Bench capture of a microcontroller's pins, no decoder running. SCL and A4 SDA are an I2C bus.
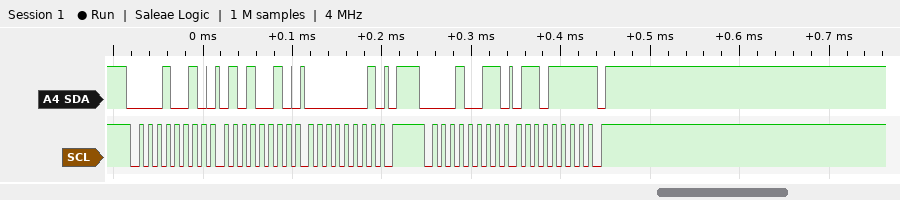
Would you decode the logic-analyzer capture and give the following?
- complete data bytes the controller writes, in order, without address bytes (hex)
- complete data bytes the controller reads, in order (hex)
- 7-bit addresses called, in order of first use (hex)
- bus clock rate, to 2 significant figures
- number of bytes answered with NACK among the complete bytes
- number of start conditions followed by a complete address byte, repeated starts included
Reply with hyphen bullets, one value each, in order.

- 52 01
- 6F
- 0x09
- 100 kHz
- 1
- 2
